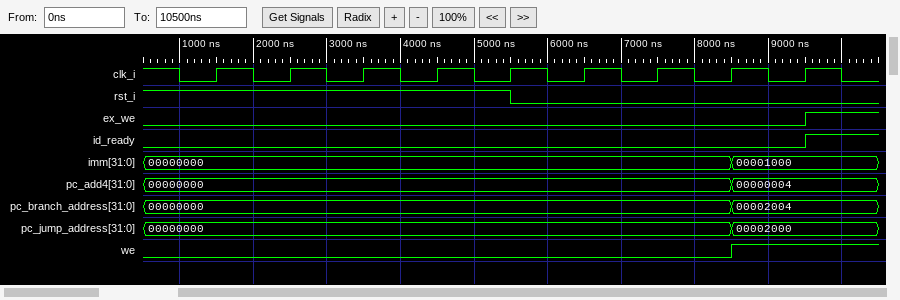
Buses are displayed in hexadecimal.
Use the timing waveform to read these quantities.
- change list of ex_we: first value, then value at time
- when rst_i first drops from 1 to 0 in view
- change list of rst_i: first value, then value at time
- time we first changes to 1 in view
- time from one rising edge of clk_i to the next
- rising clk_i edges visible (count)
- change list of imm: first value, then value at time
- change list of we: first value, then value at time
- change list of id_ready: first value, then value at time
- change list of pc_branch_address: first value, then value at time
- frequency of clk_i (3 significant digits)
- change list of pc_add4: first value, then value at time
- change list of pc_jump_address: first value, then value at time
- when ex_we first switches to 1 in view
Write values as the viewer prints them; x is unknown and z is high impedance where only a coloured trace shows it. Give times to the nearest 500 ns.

0, 1 at 9500 ns
5500 ns
1, 0 at 5500 ns
8500 ns
1000 ns
9
00000000, 00001000 at 8500 ns
0, 1 at 8500 ns
0, 1 at 9500 ns
00000000, 00002004 at 8500 ns
1.00 MHz
00000000, 00000004 at 8500 ns
00000000, 00002000 at 8500 ns
9500 ns
